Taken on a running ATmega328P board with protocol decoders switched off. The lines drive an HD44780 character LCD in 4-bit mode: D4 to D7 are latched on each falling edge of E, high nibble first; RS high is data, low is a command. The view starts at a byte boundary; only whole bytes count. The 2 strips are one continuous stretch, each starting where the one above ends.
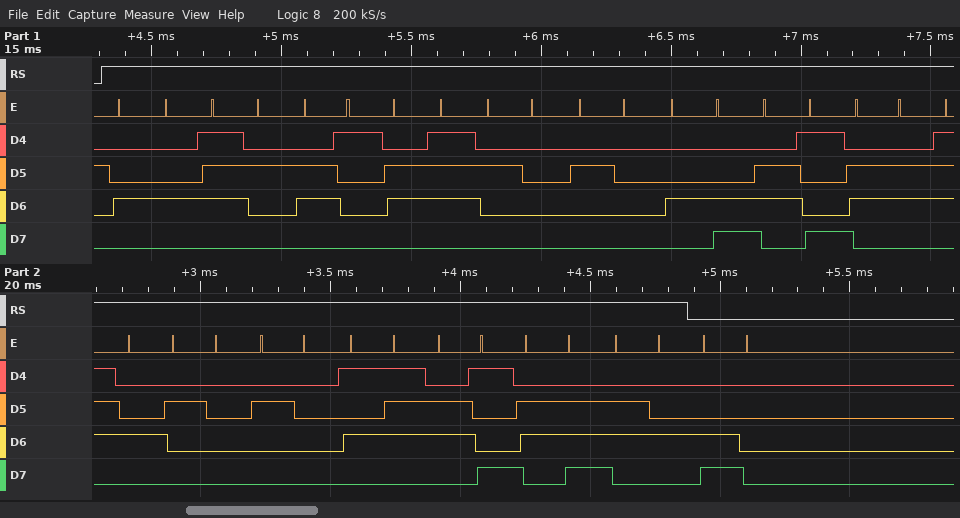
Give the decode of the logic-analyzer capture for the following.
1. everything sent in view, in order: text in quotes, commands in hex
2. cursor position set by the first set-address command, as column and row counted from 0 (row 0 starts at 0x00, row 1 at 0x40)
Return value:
"Drag  Lift  Wind" 0xC0
column 0, row 1
